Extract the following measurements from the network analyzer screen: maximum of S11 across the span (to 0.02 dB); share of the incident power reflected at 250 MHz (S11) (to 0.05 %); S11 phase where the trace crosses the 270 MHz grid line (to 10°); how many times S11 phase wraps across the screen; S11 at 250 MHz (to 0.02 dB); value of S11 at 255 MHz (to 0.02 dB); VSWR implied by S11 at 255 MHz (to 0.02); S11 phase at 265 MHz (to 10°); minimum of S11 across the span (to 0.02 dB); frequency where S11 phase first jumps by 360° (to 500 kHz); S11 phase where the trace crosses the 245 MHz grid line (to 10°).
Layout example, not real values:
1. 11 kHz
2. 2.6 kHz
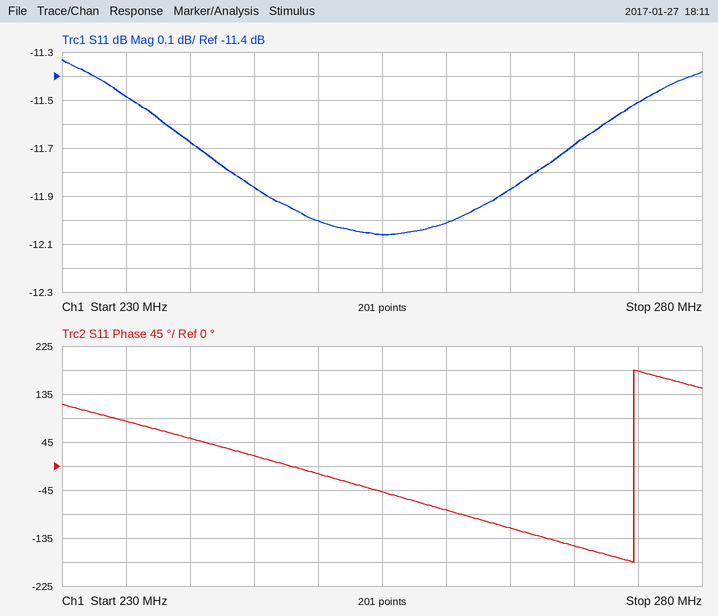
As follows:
1. -11.34 dB
2. 6.30 %
3. -150°
4. 1
5. -12.00 dB
6. -12.06 dB
7. 1.66
8. -120°
9. -12.06 dB
10. 274.5 MHz
11. 20°
